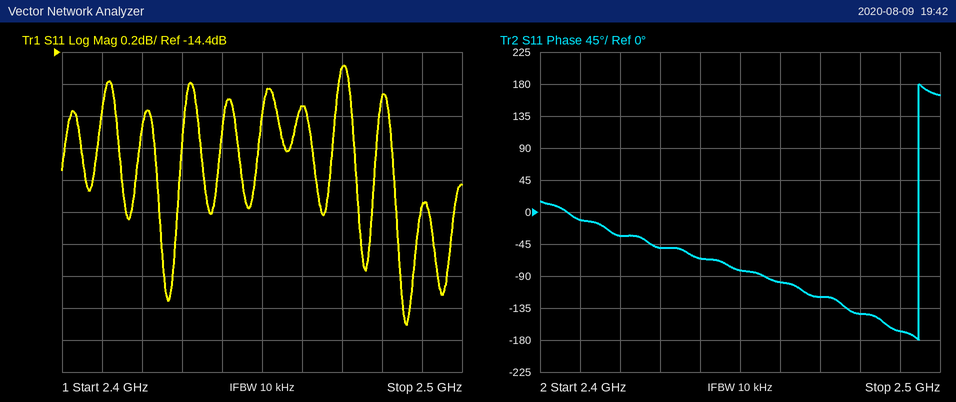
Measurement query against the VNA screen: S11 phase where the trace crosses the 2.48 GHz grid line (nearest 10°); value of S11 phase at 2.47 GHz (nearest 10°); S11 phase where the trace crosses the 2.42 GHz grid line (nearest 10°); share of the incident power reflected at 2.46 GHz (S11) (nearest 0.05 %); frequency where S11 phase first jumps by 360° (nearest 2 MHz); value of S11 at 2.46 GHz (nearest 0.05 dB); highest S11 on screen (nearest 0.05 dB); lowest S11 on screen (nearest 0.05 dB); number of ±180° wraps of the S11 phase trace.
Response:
-140°
-120°
-30°
3.35 %
2.494 GHz
-14.75 dB
-14.50 dB
-16.10 dB
1
